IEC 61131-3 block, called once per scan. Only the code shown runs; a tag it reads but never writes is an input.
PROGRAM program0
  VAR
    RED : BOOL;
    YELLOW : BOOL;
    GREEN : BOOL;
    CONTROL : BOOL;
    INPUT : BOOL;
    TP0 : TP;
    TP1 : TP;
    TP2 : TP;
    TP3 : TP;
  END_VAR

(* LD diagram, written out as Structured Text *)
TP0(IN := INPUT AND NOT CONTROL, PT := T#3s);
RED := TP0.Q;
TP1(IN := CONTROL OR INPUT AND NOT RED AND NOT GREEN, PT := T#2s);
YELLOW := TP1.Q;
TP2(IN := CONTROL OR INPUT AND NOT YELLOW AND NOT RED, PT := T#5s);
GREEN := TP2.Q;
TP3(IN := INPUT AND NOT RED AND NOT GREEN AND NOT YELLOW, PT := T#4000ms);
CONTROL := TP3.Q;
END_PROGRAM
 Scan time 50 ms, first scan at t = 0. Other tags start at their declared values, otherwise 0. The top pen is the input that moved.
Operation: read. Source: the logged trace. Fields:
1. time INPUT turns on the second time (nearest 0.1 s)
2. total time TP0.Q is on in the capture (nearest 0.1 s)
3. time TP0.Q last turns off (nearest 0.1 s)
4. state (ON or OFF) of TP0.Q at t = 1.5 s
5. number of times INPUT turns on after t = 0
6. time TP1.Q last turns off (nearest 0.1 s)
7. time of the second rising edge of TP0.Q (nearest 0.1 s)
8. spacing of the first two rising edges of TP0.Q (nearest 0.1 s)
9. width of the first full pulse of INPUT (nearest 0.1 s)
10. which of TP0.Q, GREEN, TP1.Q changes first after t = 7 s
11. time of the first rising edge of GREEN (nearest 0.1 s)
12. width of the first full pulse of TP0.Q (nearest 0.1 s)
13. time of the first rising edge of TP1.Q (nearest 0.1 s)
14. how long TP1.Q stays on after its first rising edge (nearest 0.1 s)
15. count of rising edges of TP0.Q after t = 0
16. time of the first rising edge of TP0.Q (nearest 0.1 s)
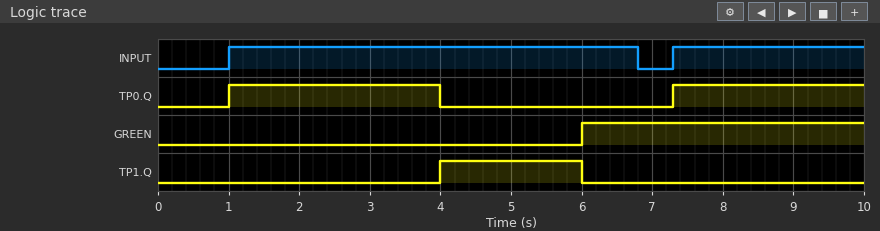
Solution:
7.3 s
5.7 s
4.0 s
ON
2
6.0 s
7.3 s
6.3 s
5.8 s
TP0.Q
6.0 s
3.0 s
4.0 s
2.0 s
2
1.0 s
